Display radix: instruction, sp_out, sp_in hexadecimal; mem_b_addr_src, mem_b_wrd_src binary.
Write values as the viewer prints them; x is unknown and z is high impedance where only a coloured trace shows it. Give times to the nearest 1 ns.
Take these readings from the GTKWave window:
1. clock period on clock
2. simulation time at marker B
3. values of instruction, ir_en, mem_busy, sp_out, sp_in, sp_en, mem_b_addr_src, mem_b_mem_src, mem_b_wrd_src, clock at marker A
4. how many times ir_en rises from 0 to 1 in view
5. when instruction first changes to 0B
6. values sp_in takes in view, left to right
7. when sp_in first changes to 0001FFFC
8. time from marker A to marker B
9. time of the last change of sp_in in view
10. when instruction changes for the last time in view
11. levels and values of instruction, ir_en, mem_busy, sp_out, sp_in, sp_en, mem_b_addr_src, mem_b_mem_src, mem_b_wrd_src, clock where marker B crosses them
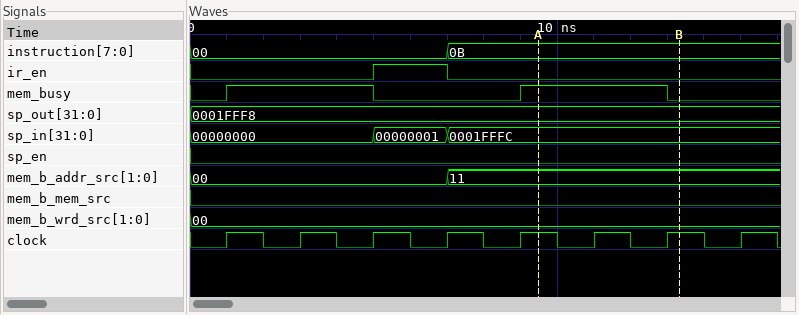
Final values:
2 ns
13 ns
instruction=0B, ir_en=0, mem_busy=1, sp_out=0001FFF8, sp_in=0001FFFC, sp_en=0, mem_b_addr_src=11, mem_b_mem_src=0, mem_b_wrd_src=00, clock=1
1
7 ns
00000000, 00000001, 0001FFFC
7 ns
4 ns
7 ns
7 ns
instruction=0B, ir_en=0, mem_busy=0, sp_out=0001FFF8, sp_in=0001FFFC, sp_en=0, mem_b_addr_src=11, mem_b_mem_src=0, mem_b_wrd_src=00, clock=1
